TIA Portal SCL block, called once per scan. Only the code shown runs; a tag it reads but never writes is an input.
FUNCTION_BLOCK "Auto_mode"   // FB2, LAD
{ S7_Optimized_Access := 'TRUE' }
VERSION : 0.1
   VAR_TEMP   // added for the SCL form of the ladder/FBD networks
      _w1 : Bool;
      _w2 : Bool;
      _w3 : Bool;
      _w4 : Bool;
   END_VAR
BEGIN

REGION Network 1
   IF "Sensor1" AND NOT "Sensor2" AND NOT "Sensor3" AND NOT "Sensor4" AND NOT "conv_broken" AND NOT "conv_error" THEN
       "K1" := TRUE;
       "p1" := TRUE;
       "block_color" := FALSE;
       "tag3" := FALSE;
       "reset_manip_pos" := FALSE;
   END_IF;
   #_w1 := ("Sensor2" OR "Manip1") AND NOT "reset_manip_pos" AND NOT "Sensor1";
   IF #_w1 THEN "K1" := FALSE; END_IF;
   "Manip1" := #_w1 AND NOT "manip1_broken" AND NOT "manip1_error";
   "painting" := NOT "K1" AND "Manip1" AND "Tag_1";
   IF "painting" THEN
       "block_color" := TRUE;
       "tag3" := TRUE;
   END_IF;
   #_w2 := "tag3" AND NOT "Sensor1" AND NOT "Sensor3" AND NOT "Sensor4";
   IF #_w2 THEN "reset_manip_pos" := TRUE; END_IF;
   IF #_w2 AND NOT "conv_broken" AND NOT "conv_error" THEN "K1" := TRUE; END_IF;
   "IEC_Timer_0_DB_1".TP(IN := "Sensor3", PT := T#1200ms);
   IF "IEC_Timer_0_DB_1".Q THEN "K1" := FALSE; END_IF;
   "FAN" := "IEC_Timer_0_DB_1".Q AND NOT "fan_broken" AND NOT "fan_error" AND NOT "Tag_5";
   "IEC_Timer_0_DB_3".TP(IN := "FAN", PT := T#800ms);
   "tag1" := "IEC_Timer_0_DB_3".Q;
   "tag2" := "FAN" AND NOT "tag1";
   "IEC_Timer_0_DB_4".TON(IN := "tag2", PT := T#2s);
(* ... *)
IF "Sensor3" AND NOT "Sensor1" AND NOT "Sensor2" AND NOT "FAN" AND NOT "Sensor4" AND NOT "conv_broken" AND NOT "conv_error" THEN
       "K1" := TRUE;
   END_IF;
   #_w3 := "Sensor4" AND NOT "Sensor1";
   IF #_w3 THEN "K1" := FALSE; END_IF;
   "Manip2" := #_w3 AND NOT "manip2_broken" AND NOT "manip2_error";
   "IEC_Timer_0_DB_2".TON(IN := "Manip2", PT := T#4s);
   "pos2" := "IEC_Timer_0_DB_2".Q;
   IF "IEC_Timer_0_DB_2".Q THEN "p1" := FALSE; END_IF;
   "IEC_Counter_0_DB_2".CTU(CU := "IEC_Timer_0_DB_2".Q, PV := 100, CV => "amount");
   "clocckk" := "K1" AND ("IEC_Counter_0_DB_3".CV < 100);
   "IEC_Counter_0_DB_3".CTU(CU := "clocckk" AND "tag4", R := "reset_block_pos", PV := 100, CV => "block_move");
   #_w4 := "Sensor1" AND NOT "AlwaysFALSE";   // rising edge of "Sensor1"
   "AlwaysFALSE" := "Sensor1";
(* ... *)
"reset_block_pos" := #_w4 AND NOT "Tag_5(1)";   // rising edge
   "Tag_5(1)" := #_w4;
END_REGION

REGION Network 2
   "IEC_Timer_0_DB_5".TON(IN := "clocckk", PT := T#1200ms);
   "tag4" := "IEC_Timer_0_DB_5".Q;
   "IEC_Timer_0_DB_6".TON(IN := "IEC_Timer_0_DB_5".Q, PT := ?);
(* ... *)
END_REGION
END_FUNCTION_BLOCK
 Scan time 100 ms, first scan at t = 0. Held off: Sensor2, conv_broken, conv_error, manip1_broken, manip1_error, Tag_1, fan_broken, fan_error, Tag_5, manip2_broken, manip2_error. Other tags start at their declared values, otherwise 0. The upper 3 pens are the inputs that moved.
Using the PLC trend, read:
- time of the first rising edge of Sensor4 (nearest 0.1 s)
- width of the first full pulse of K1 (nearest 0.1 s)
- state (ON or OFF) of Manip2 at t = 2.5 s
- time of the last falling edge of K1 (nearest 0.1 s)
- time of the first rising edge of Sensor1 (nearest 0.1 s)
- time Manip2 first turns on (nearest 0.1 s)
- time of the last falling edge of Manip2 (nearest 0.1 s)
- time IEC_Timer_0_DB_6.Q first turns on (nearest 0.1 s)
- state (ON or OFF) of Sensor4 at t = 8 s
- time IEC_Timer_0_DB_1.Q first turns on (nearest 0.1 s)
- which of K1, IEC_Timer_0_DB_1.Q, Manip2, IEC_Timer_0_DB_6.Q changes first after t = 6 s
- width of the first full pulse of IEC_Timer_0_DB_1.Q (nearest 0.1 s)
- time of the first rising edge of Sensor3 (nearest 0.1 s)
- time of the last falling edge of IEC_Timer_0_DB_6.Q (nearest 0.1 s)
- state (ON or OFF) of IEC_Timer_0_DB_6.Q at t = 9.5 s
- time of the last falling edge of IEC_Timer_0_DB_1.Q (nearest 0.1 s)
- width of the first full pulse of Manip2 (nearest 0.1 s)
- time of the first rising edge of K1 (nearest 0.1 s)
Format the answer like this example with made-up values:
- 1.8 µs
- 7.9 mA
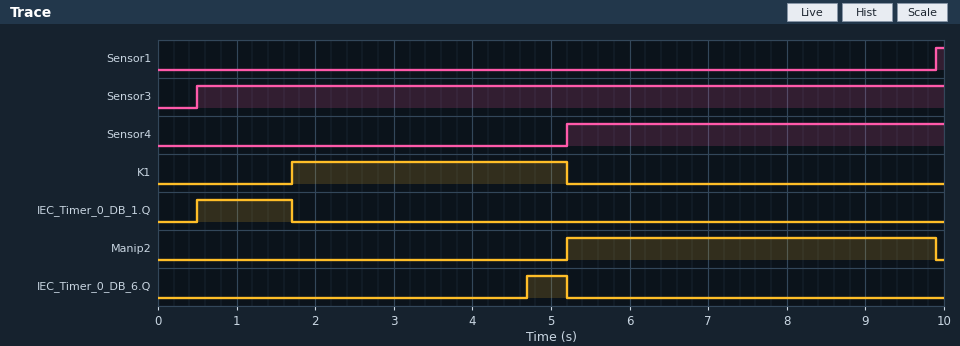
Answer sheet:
- 5.2 s
- 3.5 s
- OFF
- 5.2 s
- 9.9 s
- 5.2 s
- 9.9 s
- 4.7 s
- ON
- 0.5 s
- Manip2
- 1.2 s
- 0.5 s
- 5.2 s
- OFF
- 1.7 s
- 4.7 s
- 1.7 s
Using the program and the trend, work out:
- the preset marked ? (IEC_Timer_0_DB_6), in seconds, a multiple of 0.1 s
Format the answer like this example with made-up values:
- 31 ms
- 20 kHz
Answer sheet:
- 1.8 s
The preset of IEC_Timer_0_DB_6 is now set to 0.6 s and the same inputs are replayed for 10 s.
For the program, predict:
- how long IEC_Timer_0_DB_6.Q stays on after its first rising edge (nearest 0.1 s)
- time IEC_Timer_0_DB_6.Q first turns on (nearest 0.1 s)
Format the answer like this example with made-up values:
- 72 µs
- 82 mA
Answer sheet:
- 1.7 s
- 3.5 s
